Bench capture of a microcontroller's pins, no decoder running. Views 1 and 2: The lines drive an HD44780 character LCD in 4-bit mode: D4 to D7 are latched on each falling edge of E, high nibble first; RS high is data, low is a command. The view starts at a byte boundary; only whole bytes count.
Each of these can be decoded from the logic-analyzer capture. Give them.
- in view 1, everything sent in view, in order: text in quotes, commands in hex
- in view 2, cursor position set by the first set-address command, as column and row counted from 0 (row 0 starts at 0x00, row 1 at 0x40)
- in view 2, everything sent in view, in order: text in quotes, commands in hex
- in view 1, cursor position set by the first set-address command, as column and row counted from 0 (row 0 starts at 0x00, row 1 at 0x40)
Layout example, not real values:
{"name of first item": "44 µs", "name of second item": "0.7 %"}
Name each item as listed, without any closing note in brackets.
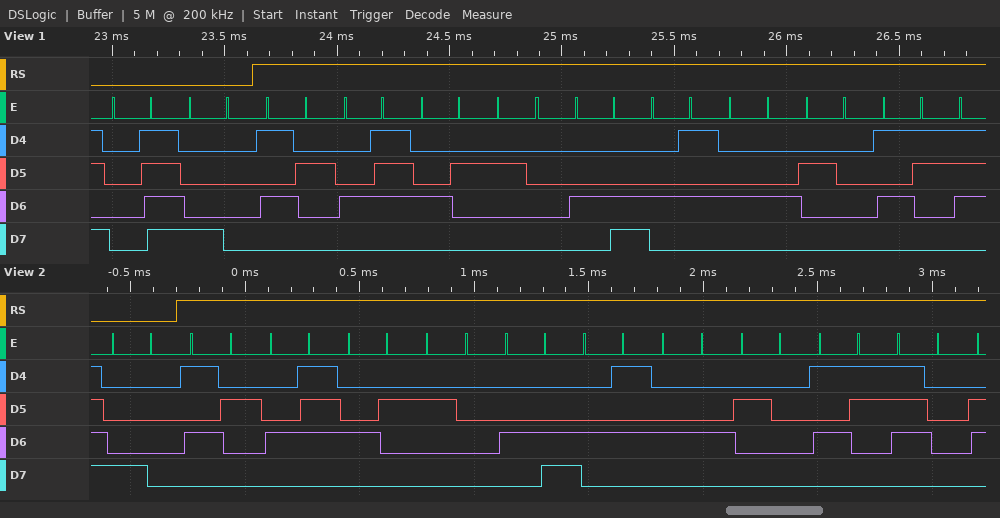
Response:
{"in view 1, everything sent in view, in order: text in quotes, commands in hex": "0x0F 0x80 \"RGB LED S\"", "in view 2, cursor position set by the first set-address command, as column and row counted from 0": "column 0, row 0", "in view 2, everything sent in view, in order: text in quotes, commands in hex": "0x80 \"RGB LED Sp\"", "in view 1, cursor position set by the first set-address command, as column and row counted from 0": "column 0, row 0"}
